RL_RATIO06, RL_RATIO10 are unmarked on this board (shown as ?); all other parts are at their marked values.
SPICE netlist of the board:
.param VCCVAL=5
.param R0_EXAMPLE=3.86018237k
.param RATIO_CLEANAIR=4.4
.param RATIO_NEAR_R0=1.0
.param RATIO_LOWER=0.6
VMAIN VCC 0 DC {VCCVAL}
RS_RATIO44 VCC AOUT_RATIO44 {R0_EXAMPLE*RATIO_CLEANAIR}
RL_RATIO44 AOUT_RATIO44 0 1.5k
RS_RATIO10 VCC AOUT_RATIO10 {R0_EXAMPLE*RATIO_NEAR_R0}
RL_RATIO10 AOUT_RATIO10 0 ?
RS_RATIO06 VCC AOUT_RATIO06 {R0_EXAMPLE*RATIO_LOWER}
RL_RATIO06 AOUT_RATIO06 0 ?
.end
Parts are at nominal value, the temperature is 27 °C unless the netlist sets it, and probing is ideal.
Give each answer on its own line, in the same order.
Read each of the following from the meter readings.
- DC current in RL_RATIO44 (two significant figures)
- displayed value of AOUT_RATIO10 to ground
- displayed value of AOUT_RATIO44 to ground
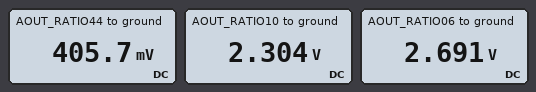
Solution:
270 µA
2.304 V
405.7 mV
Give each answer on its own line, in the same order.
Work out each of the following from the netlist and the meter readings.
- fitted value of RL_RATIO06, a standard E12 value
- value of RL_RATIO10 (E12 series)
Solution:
2.7 kΩ
3.3 kΩ
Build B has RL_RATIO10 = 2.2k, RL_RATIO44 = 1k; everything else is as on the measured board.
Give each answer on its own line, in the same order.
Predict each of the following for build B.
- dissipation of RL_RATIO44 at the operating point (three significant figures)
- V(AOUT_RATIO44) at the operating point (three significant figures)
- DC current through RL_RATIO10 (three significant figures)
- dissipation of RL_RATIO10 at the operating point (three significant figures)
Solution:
77.3 µW
278 mV
825 µA
1.50 mW
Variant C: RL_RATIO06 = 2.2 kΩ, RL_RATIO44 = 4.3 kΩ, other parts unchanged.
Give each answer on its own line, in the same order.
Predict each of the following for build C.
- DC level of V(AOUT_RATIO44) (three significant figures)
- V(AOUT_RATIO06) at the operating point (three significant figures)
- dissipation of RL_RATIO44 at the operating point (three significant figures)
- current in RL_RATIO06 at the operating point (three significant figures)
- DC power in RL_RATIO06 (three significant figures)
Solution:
1.01 V
2.44 V
237 µW
1.11 mA
2.70 mW
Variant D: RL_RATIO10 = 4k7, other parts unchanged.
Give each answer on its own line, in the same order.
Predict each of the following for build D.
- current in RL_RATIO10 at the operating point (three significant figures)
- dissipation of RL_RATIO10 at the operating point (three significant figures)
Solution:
584 µA
1.60 mW
